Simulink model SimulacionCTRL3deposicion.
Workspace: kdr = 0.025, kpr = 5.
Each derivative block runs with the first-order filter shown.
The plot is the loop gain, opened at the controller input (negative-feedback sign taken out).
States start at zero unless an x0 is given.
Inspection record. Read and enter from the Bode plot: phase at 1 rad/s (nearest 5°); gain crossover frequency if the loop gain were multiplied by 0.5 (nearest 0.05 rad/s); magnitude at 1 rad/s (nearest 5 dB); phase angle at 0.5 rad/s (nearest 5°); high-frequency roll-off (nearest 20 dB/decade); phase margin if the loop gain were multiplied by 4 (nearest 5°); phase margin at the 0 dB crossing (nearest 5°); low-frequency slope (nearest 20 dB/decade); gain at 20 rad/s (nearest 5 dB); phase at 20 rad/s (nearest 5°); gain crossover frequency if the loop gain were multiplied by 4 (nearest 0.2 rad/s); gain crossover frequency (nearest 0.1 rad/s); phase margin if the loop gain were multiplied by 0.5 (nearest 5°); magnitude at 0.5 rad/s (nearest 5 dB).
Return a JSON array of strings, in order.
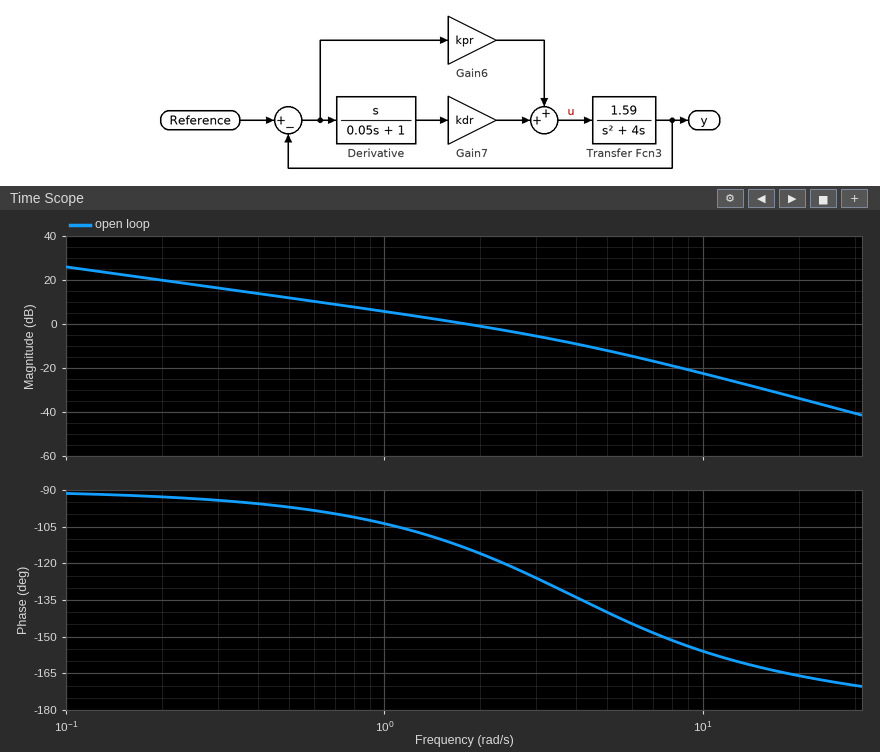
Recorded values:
["-105°", "0.95 rad/s", "5 dB", "-95°", "-40 dB/decade", "40°", "65°", "-20 dB/decade", "-35 dB", "-165°", "5.0 rad/s", "1.8 rad/s", "75°", "10 dB"]
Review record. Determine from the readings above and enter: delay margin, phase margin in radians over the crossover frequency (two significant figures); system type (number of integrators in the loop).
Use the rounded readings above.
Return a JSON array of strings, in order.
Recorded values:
["0.63 s", "1"]
